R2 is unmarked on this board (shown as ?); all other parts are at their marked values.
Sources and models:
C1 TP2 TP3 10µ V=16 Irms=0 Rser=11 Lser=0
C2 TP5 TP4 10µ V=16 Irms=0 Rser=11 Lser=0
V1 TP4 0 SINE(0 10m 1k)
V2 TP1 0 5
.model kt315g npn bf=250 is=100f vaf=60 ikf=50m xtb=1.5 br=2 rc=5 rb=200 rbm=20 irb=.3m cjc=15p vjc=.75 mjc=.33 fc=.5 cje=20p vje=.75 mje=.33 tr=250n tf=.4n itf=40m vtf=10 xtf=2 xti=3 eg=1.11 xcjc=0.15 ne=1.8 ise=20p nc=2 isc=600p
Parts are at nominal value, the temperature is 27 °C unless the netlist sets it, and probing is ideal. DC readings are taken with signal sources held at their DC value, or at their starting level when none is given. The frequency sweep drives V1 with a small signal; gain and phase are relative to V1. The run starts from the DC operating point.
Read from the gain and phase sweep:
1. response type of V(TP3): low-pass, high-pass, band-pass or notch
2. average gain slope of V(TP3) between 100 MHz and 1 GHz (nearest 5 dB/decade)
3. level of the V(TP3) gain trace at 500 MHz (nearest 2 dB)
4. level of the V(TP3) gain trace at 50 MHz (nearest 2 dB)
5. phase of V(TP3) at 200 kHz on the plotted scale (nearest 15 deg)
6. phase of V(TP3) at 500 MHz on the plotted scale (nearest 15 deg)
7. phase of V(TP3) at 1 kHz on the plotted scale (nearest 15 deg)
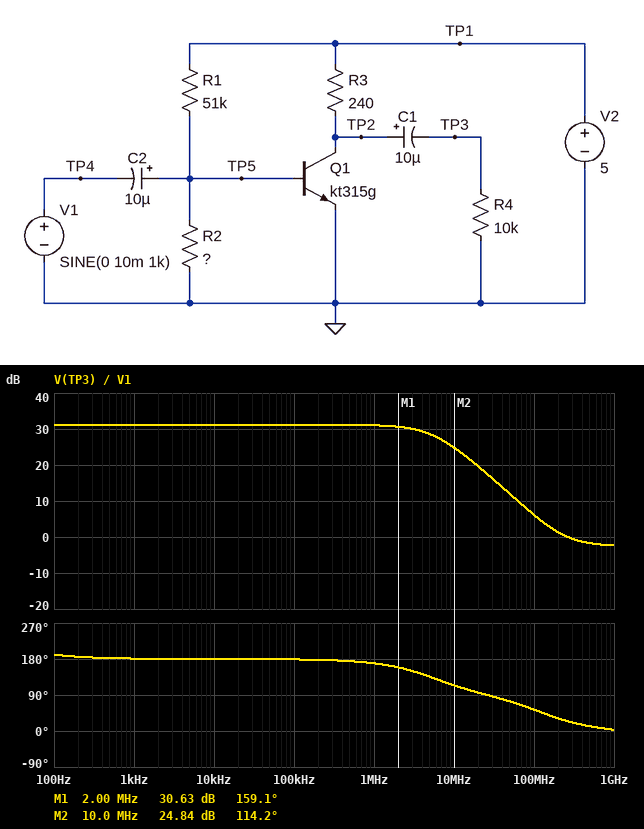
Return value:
low-pass
-10 dB/decade
-2 dB
12 dB
180 deg
15 deg
180 deg
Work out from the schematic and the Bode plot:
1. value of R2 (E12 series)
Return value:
15 kΩ
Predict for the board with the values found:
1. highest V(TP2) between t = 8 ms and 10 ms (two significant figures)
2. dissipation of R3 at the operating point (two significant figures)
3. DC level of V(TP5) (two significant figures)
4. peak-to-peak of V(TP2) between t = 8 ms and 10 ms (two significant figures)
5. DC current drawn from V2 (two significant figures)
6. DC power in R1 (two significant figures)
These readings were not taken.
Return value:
4.0 V
7.2 mW
650 mV
740 mV
5.6 mA
370 µW
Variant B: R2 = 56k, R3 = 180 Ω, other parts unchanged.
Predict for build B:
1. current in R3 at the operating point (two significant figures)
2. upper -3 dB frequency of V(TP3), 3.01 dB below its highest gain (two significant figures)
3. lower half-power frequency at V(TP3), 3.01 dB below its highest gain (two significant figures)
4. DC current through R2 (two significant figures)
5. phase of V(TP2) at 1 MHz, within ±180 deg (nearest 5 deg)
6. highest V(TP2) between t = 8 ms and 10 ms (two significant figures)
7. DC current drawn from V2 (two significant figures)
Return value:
9.9 mA
4.4 MHz
28 Hz
12 µA
165 deg
3.6 V
10 mA
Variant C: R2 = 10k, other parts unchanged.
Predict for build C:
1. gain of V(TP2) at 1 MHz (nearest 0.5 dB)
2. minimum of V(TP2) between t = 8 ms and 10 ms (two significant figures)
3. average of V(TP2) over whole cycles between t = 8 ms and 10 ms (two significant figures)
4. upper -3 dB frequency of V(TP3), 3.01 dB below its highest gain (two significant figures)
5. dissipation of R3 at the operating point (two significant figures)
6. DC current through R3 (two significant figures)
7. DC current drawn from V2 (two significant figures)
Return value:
26.0 dB
4.1 V
4.3 V
8.2 MHz
1.8 mW
2.7 mA
2.8 mA
